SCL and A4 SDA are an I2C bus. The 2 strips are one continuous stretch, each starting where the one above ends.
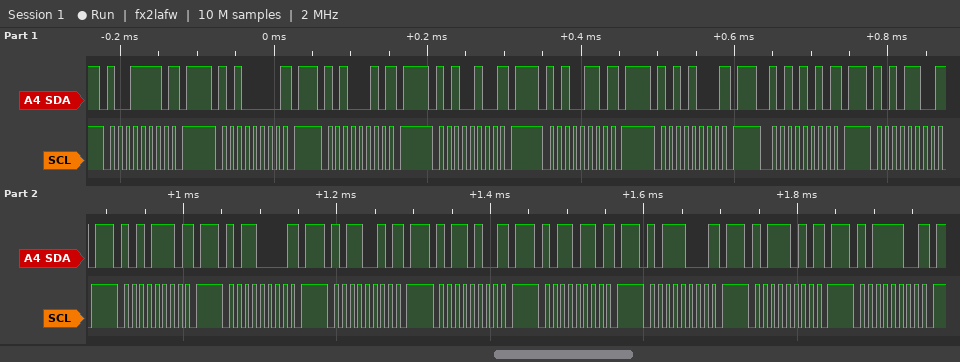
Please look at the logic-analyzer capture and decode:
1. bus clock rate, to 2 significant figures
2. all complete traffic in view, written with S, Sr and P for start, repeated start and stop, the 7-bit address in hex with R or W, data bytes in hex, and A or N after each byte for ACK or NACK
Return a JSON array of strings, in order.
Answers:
["100 kHz", "S 4FW N P S 50W N P S 51W N P S 52W N P S 53W N P S 54W N P S 55W N P S 56W N P S 57W N P S 58W N P S 59W N P S 5AW N P S 5BW N P S 5CW N P S 5DW N P S 5EW N P"]
